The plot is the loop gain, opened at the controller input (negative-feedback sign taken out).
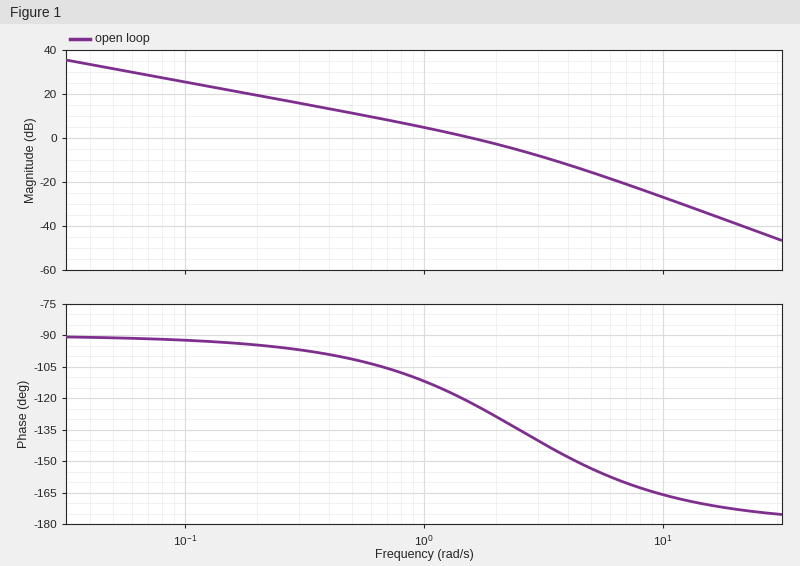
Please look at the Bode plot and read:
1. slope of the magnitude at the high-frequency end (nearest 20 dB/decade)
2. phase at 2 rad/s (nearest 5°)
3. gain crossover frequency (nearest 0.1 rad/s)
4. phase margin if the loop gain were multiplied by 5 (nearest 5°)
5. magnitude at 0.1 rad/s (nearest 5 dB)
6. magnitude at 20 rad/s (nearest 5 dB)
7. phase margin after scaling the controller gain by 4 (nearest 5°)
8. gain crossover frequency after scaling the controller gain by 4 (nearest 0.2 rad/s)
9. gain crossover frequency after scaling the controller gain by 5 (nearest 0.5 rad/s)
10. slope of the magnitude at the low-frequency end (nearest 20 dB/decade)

-40 dB/decade
-130°
1.6 rad/s
30°
25 dB
-40 dB
30°
4.0 rad/s
4.5 rad/s
-20 dB/decade
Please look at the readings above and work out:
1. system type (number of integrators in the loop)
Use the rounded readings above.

1
